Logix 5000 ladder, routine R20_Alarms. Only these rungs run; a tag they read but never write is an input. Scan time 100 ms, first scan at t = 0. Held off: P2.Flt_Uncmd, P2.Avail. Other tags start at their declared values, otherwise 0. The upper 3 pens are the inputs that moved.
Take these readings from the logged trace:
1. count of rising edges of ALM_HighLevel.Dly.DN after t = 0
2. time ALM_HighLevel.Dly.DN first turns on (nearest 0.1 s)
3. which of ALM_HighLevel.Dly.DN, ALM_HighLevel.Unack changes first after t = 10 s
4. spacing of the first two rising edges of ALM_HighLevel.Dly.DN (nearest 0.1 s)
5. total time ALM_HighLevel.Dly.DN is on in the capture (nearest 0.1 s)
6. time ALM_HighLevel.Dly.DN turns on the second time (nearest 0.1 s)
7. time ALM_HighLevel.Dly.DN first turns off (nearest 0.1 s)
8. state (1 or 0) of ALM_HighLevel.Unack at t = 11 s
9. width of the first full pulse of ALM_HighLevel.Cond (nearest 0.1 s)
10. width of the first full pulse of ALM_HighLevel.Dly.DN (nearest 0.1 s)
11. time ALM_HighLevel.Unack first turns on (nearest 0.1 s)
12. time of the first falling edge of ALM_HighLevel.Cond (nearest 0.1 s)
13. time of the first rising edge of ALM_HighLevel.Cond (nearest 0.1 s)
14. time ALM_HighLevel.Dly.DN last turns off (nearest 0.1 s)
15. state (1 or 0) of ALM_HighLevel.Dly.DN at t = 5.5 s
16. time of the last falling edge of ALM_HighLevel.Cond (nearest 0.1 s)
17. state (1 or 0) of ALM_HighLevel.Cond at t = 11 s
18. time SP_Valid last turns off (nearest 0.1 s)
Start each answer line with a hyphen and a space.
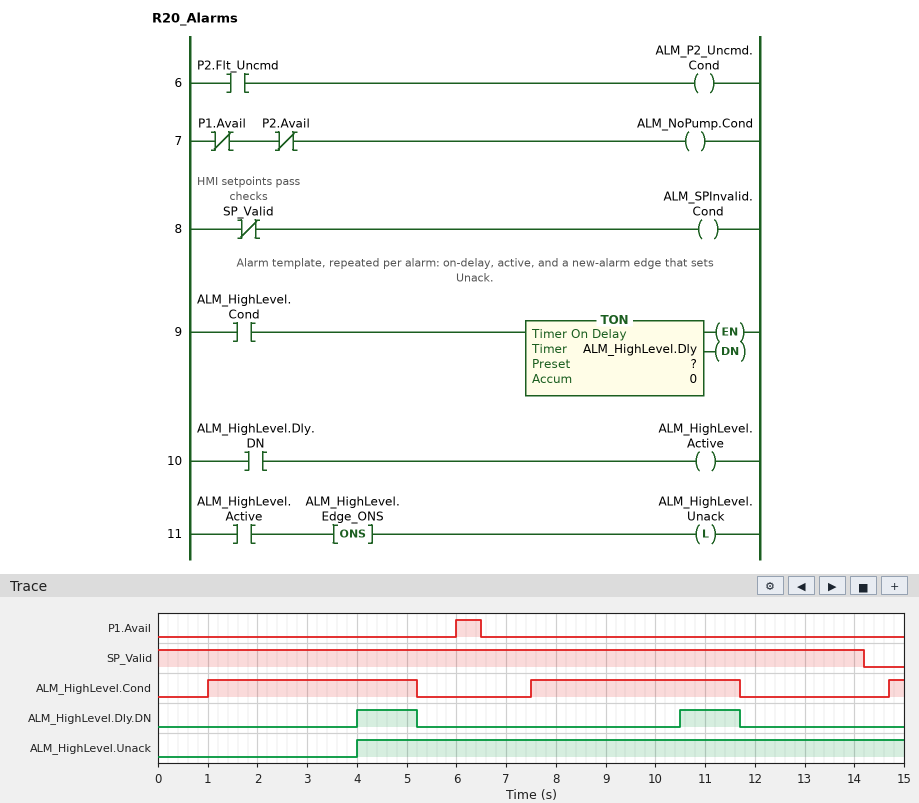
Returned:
- 2
- 4.0 s
- ALM_HighLevel.Dly.DN
- 6.5 s
- 2.4 s
- 10.5 s
- 5.2 s
- 1
- 4.2 s
- 1.2 s
- 4.0 s
- 5.2 s
- 1.0 s
- 11.7 s
- 0
- 11.7 s
- 1
- 14.2 s
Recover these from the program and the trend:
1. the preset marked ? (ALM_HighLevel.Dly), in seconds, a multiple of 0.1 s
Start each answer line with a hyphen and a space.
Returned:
- 3.0 s
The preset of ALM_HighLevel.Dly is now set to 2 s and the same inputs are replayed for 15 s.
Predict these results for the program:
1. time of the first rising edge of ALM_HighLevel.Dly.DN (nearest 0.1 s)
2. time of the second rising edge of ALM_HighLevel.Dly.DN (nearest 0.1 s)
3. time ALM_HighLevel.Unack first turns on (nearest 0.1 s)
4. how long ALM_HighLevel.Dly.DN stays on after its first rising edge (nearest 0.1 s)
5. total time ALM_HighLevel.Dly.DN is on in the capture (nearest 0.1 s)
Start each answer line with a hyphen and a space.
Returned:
- 3.0 s
- 9.5 s
- 3.0 s
- 2.2 s
- 4.4 s
